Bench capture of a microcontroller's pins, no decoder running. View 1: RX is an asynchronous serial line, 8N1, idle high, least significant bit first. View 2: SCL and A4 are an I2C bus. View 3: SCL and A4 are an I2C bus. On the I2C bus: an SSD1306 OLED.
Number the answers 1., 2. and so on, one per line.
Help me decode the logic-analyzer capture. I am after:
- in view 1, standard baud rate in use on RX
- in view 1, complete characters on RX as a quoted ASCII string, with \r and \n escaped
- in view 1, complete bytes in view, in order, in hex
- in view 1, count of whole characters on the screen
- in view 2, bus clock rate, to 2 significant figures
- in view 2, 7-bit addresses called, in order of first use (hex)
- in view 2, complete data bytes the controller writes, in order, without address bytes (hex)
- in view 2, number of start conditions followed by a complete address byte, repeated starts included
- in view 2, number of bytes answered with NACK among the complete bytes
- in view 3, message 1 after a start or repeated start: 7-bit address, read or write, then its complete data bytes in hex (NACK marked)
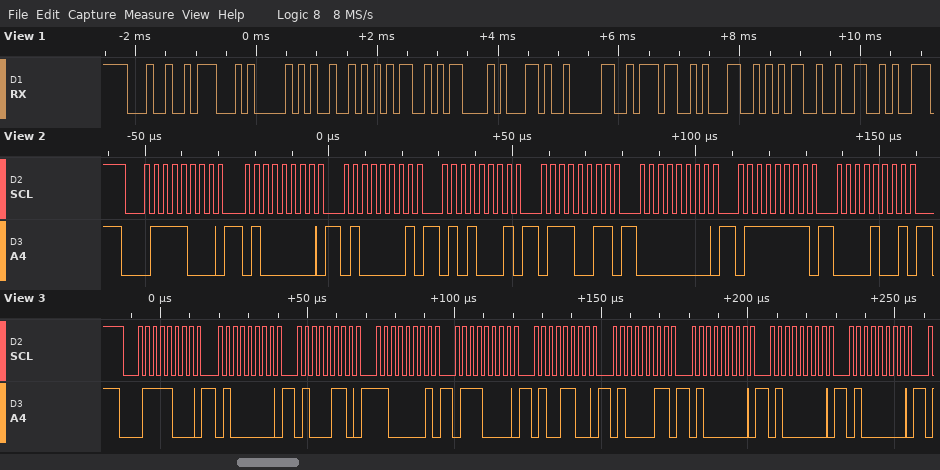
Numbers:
1. 9600 baud
2. "$GPRMC,07152"
3. 24 47 50 52 4D 43 2C 30 37 31 35 32
4. 12
5. 400 kHz
6. 0x3C
7. 40 41 51 73 00 7F 09
8. 1
9. 0
10. 0x3C write: 40 46 C1 70 4C 43 40 40 40
